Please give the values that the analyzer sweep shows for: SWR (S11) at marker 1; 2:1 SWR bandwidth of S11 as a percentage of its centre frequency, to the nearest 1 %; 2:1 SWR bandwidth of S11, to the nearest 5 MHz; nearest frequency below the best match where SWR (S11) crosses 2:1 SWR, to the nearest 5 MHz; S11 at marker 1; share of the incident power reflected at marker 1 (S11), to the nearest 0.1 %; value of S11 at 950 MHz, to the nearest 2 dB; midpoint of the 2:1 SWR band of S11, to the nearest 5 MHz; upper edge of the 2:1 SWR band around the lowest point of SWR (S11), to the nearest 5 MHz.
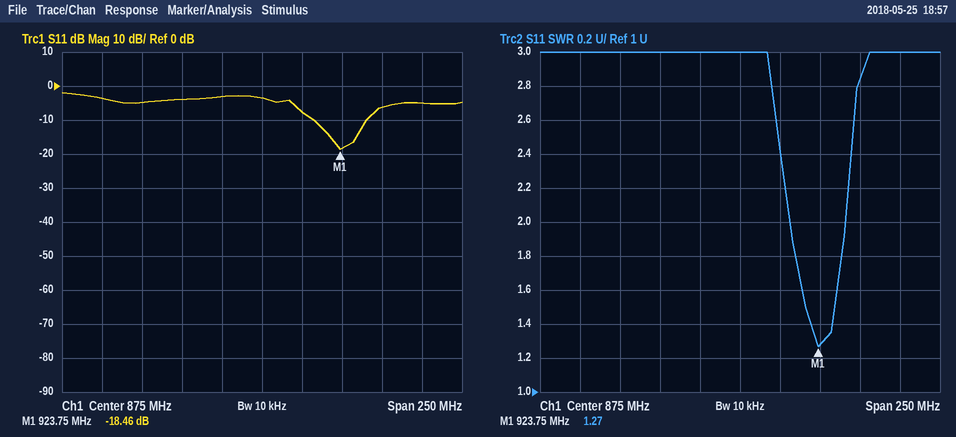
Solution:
1.27
4 %
35 MHz
905 MHz
-18.46 dB
1.4 %
-6 dB
925 MHz
940 MHz
